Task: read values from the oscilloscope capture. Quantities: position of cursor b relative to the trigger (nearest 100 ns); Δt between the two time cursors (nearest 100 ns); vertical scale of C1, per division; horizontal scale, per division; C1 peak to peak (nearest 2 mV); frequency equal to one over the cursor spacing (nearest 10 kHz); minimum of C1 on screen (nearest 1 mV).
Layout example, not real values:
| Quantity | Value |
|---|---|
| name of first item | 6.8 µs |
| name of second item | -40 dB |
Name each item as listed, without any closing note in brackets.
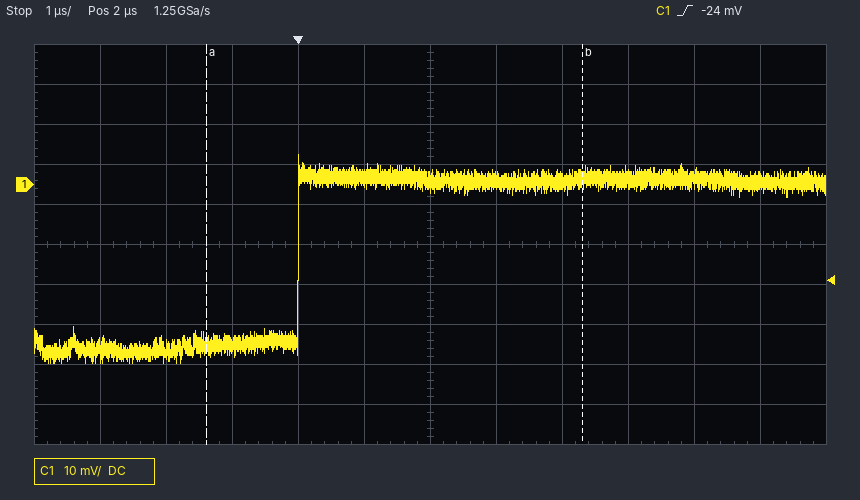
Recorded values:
| Quantity | Value |
|---|---|
| position of cursor b relative to the trigger | +4.3 µs |
| Δt between the two time cursors | 5.7 µs |
| vertical scale of C1, per division | 10 mV |
| horizontal scale, per division | 1 µs |
| C1 peak to peak | 52 mV |
| frequency equal to one over the cursor spacing | 180 kHz |
| minimum of C1 on screen | -45 mV |
